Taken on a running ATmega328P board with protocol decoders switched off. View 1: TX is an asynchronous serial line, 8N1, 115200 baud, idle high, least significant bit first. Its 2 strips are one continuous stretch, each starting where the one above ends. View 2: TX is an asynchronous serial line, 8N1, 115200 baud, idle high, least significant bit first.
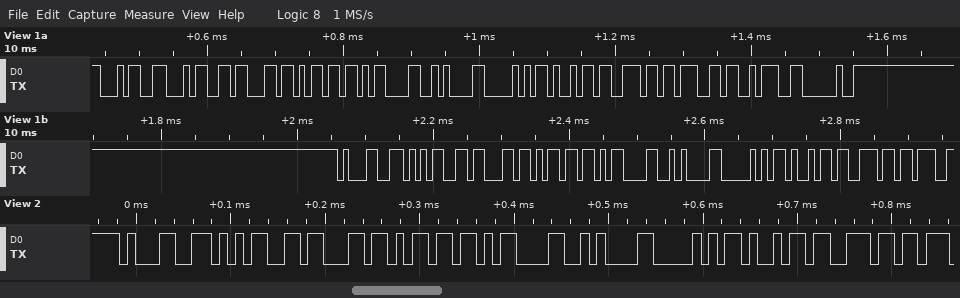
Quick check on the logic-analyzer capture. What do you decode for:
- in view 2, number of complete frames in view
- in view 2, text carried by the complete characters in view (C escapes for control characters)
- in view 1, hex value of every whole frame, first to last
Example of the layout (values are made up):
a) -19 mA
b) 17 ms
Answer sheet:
a) 9
b) "15cm\r\nPin"
c) 34 34 63 6D 0D 0A 50 69 6E 67 3A 20 31 35 63 6D 0D 0A 50 69 6E
